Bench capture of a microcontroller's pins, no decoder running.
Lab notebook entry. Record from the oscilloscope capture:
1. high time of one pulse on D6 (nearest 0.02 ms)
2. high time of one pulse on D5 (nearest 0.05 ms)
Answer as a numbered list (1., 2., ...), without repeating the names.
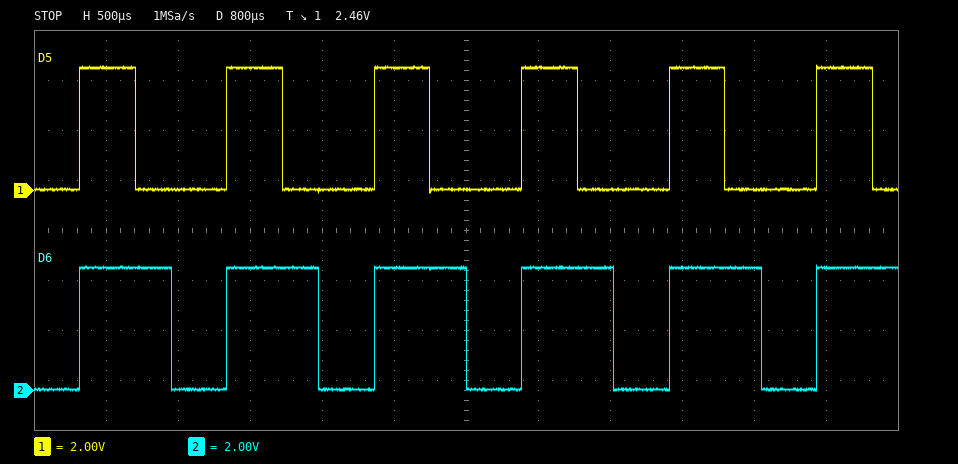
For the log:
1. 0.64 ms
2. 0.40 ms
